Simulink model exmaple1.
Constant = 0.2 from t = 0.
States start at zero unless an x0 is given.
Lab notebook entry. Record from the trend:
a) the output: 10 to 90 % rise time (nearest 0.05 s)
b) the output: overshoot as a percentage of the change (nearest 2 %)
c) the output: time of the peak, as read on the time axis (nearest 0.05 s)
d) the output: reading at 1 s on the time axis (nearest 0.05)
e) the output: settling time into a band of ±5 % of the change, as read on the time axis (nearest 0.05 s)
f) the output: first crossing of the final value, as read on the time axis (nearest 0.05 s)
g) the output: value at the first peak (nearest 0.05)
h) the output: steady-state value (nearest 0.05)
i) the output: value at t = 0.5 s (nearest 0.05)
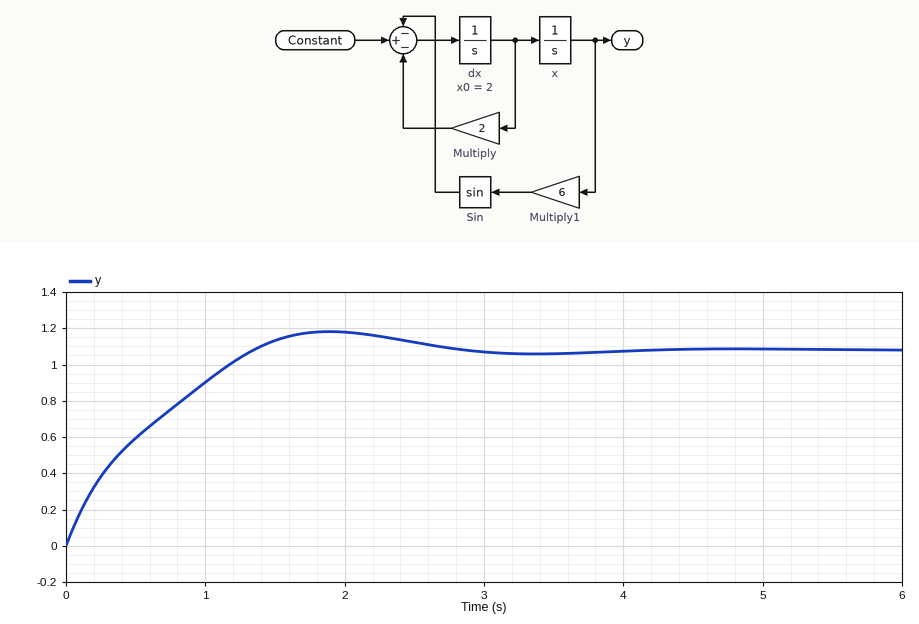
1.05 s
10 %
1.90 s
0.90
2.40 s
1.35 s
1.20
1.10
0.60
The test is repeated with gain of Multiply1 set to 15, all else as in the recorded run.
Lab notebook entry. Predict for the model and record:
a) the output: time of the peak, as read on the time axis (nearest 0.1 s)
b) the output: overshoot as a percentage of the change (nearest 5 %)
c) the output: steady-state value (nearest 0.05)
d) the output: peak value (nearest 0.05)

1.3 s
15 %
0.85
0.95
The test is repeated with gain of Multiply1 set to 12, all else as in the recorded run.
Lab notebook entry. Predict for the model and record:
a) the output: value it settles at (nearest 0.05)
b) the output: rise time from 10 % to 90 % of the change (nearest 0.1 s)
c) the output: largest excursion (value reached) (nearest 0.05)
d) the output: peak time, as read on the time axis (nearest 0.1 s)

1.05
1.2 s
1.15
1.9 s
